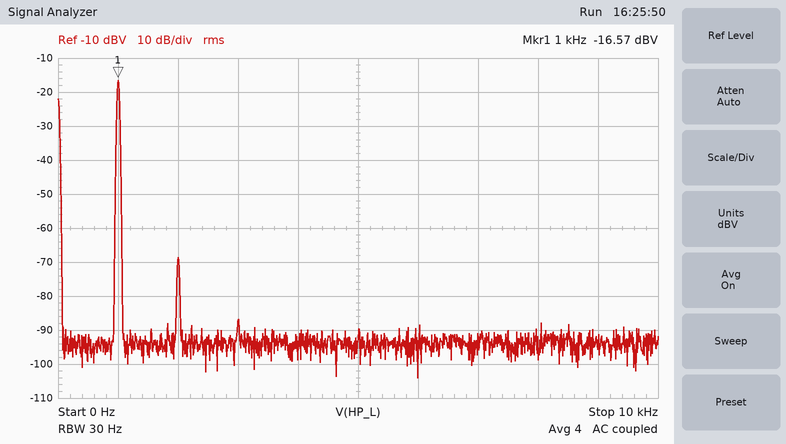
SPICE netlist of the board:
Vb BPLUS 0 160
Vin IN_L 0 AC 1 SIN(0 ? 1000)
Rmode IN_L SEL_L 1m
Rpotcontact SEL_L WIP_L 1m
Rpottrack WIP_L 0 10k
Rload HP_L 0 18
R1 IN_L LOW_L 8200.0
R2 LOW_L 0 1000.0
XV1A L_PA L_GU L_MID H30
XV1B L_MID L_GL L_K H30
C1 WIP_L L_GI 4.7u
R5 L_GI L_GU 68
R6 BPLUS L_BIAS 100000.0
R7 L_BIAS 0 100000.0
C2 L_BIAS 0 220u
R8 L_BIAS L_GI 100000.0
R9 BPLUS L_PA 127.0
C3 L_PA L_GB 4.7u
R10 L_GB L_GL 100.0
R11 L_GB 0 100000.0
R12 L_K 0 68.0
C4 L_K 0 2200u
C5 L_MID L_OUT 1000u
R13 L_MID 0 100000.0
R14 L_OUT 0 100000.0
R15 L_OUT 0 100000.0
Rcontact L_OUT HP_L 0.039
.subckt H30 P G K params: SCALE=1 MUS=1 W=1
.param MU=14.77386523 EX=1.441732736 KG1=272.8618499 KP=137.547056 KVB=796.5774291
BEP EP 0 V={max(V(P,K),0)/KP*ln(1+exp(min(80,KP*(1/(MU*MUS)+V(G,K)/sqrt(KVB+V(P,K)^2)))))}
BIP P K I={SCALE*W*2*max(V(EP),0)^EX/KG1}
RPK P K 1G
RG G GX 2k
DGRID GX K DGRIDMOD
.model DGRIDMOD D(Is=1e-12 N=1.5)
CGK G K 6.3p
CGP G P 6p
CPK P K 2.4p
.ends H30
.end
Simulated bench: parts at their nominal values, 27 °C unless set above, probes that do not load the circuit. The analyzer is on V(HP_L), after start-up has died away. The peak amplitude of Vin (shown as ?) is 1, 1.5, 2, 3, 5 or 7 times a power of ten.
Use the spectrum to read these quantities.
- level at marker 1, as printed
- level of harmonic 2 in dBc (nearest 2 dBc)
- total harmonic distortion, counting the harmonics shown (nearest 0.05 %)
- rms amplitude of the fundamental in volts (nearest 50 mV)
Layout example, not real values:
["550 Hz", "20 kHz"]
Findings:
["-16.57 dBV", "-52 dBc", "0.25 %", "150 mV"]
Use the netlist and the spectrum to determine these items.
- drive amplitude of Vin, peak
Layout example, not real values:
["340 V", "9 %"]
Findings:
["500 mV"]
